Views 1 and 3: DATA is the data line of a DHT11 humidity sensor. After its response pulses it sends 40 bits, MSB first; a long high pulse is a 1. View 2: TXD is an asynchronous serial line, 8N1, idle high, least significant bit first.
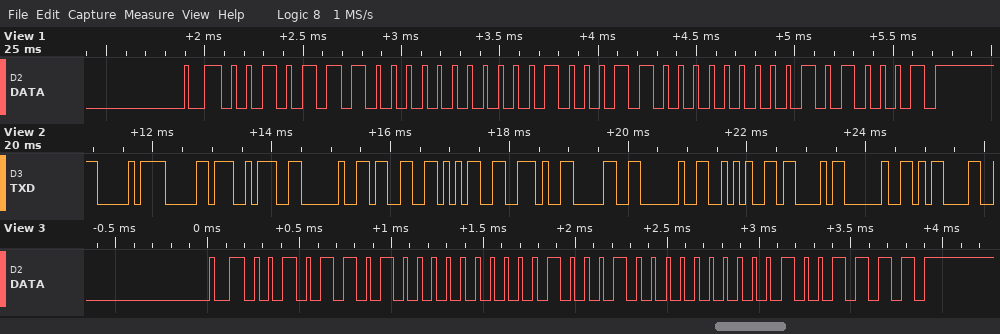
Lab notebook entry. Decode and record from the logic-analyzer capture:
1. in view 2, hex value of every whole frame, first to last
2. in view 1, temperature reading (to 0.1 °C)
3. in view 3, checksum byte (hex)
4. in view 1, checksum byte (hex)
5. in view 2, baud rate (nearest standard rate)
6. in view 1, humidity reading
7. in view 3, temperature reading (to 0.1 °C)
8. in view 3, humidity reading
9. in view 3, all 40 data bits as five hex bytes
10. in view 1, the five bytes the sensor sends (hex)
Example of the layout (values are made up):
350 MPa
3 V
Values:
D0 B0 3A 20 33 35 2E 30 20 2A 43 20 0D
35.0 °C
0x4F
0x51
9600 baud
46 %
34.0 °C
45 %
2D 00 22 00 4F
2E 00 23 00 51
